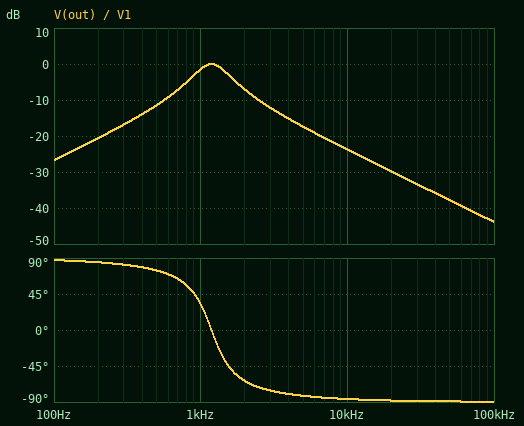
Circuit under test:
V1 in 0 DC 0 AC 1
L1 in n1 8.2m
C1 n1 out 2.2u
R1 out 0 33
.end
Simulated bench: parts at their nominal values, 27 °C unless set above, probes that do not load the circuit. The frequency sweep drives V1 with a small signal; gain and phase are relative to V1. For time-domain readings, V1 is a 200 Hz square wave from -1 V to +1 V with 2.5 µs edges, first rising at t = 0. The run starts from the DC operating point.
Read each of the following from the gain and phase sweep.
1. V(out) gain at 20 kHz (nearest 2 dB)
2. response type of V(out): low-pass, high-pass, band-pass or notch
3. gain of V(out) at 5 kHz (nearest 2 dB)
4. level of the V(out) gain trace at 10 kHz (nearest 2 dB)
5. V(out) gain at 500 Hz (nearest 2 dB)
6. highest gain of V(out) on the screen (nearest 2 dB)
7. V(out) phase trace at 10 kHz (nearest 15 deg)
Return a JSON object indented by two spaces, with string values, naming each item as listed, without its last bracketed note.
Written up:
{
  "V(out) gain at 20 kHz": "-30 dB",
  "response type of V(out): low-pass, high-pass, band-pass or notch": "band-pass",
  "gain of V(out) at 5 kHz": "-18 dB",
  "level of the V(out) gain trace at 10 kHz": "-24 dB",
  "V(out) gain at 500 Hz": "-12 dB",
  "highest gain of V(out) on the screen": "0 dB",
  "V(out) phase trace at 10 kHz": "-90 deg"
}
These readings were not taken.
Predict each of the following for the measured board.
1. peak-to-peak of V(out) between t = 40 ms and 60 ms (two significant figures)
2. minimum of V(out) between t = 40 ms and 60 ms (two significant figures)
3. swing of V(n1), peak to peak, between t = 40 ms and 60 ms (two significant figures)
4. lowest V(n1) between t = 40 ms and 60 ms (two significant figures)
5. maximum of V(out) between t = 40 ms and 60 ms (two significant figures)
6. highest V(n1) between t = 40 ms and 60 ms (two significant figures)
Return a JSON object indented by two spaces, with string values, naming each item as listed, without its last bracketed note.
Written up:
{
  "peak-to-peak of V(out) between t = 40 ms and 60 ms": "1.5 V",
  "minimum of V(out) between t = 40 ms and 60 ms": "-750 mV",
  "swing of V(n1), peak to peak, between t = 40 ms and 60 ms": "3.9 V",
  "lowest V(n1) between t = 40 ms and 60 ms": "-2.0 V",
  "maximum of V(out) between t = 40 ms and 60 ms": "750 mV",
  "highest V(n1) between t = 40 ms and 60 ms": "2.0 V"
}
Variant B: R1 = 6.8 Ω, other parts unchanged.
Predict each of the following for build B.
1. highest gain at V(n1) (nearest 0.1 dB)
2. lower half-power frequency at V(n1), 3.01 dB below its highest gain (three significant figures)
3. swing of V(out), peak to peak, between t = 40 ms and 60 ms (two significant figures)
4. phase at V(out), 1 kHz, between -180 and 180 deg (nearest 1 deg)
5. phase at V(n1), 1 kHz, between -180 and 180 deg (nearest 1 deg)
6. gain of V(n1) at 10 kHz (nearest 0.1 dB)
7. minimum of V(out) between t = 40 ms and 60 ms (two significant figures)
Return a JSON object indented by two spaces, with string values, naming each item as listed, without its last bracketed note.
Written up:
{
  "highest gain at V(n1)": "19.1 dB",
  "lower half-power frequency at V(n1), 3.01 dB below its highest gain": "1.11 kHz",
  "swing of V(out), peak to peak, between t = 40 ms and 60 ms": "310 mV",
  "phase at V(out), 1 kHz, between -180 and 180 deg": "72 deg",
  "phase at V(n1), 1 kHz, between -180 and 180 deg": "-13 deg",
  "gain of V(n1) at 10 kHz": "-34.2 dB",
  "minimum of V(out) between t = 40 ms and 60 ms": "-150 mV"
}
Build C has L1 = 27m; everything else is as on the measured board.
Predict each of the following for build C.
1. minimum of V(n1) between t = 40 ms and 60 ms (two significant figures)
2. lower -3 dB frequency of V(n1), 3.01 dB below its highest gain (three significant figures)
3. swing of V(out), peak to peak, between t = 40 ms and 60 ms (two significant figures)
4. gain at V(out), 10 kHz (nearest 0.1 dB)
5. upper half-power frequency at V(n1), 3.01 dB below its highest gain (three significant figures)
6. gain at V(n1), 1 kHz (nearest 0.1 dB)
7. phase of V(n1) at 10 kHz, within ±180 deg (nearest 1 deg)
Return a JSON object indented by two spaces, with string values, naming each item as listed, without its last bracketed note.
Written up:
{
  "minimum of V(n1) between t = 40 ms and 60 ms": "-2.6 V",
  "lower -3 dB frequency of V(n1), 3.01 dB below its highest gain": "534 Hz",
  "swing of V(out), peak to peak, between t = 40 ms and 60 ms": "1.2 V",
  "gain at V(out), 10 kHz": "-34.2 dB",
  "upper half-power frequency at V(n1), 3.01 dB below its highest gain": "732 Hz",
  "gain at V(n1), 1 kHz": "-2.2 dB",
  "phase of V(n1) at 10 kHz, within ±180 deg": "-101 deg"
}
